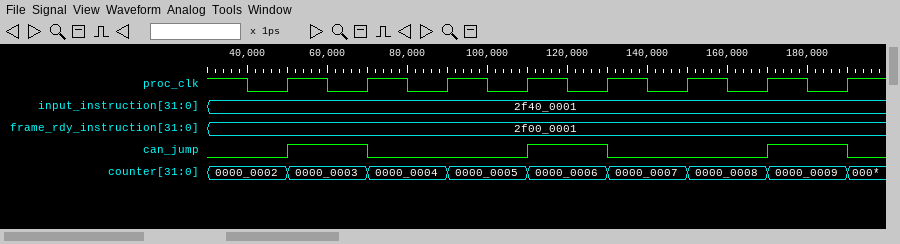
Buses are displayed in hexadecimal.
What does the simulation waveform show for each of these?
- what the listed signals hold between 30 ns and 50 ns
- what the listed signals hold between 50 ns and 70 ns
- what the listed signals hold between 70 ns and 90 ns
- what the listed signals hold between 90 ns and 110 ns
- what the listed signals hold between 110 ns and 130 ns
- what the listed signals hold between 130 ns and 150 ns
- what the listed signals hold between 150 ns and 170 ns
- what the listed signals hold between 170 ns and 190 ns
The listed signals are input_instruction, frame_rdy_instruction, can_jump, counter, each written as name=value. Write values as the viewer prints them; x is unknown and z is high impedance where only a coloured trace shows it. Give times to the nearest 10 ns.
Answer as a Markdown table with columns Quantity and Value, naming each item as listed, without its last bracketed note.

| Quantity | Value |
|---|---|
| what the listed signals hold between 30 ns and 50 ns | input_instruction=2f40_0001, frame_rdy_instruction=2f00_0001, can_jump=0, counter=0000_0002 |
| what the listed signals hold between 50 ns and 70 ns | input_instruction=2f40_0001, frame_rdy_instruction=2f00_0001, can_jump=1, counter=0000_0003 |
| what the listed signals hold between 70 ns and 90 ns | input_instruction=2f40_0001, frame_rdy_instruction=2f00_0001, can_jump=0, counter=0000_0004 |
| what the listed signals hold between 90 ns and 110 ns | input_instruction=2f40_0001, frame_rdy_instruction=2f00_0001, can_jump=0, counter=0000_0005 |
| what the listed signals hold between 110 ns and 130 ns | input_instruction=2f40_0001, frame_rdy_instruction=2f00_0001, can_jump=1, counter=0000_0006 |
| what the listed signals hold between 130 ns and 150 ns | input_instruction=2f40_0001, frame_rdy_instruction=2f00_0001, can_jump=0, counter=0000_0007 |
| what the listed signals hold between 150 ns and 170 ns | input_instruction=2f40_0001, frame_rdy_instruction=2f00_0001, can_jump=0, counter=0000_0008 |
| what the listed signals hold between 170 ns and 190 ns | input_instruction=2f40_0001, frame_rdy_instruction=2f00_0001, can_jump=1, counter=0000_0009 |
